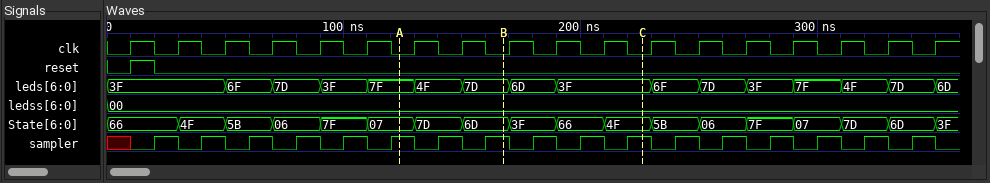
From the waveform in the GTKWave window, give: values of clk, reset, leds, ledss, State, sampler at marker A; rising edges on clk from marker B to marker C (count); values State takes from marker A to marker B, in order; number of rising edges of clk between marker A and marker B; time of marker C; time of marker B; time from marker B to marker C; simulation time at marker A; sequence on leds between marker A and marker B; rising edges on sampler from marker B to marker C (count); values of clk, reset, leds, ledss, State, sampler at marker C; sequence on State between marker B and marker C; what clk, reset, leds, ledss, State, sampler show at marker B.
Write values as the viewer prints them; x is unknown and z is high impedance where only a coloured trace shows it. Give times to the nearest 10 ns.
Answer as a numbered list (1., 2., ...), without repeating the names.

1. clk=0, reset=0, leds=7F, ledss=00, State=07, sampler=1
2. 3
3. 07, 7D, 6D
4. 2
5. 230 ns
6. 170 ns
7. 60 ns
8. 120 ns
9. 7F, 4F, 7D
10. 3
11. clk=0, reset=0, leds=3F, ledss=00, State=4F, sampler=1
12. 6D, 3F, 66, 4F
13. clk=0, reset=0, leds=7D, ledss=00, State=6D, sampler=1
